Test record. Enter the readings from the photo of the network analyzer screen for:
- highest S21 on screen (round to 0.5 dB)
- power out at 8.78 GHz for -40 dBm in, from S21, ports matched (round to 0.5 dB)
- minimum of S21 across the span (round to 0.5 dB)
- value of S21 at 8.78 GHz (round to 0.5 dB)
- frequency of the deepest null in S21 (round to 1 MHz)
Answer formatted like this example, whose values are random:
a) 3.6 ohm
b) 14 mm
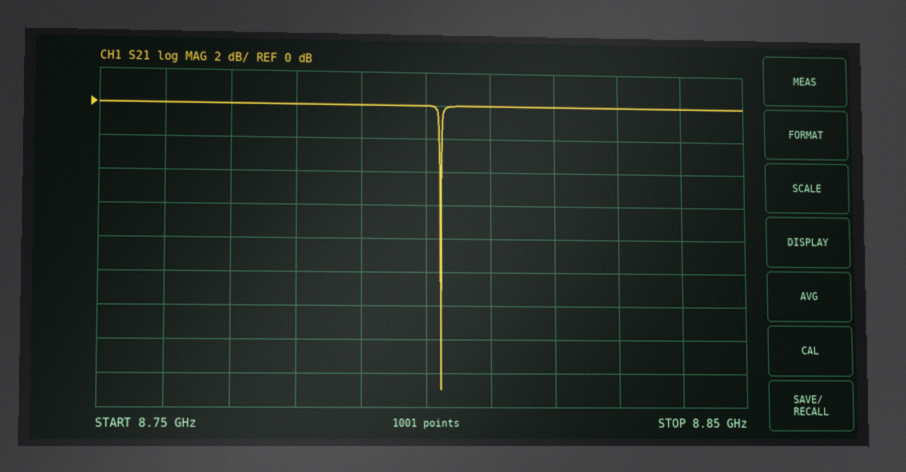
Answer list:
a) 0.0 dB
b) -40.0 dBm
c) -17.0 dB
d) 0.0 dB
e) 8.802 GHz
